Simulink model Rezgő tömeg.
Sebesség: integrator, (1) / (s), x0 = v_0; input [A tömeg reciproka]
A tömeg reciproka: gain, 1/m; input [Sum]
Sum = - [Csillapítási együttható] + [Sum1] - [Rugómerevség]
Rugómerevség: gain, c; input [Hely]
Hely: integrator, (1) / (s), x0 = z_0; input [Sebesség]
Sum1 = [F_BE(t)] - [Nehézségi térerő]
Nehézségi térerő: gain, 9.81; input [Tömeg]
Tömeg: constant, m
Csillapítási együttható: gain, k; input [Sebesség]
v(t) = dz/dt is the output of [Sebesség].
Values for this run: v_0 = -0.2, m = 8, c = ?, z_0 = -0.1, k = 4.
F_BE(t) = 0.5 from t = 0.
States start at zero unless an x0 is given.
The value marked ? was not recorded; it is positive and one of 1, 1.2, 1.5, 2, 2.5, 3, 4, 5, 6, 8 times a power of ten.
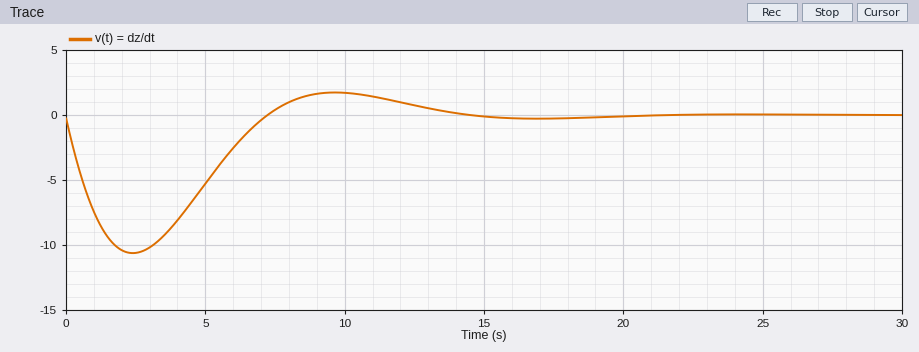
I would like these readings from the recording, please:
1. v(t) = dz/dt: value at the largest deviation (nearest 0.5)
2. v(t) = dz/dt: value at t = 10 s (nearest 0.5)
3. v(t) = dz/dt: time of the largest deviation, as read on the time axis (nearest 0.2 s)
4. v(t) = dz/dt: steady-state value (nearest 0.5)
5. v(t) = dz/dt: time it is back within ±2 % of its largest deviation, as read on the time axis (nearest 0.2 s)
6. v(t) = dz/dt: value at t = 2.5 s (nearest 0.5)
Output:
-10.5
1.5
2.4 s
0.0
18.6 s
-10.5
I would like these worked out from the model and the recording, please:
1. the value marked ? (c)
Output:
2
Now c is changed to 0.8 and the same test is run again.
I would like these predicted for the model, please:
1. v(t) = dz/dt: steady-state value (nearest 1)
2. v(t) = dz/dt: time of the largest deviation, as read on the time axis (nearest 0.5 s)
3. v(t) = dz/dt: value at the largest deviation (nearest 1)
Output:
0
3.5 s
-13
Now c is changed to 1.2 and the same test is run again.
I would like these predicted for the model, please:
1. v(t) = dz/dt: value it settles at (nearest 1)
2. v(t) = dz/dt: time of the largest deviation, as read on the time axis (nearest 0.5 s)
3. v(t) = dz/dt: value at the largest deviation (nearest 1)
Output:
0
3.0 s
-12
